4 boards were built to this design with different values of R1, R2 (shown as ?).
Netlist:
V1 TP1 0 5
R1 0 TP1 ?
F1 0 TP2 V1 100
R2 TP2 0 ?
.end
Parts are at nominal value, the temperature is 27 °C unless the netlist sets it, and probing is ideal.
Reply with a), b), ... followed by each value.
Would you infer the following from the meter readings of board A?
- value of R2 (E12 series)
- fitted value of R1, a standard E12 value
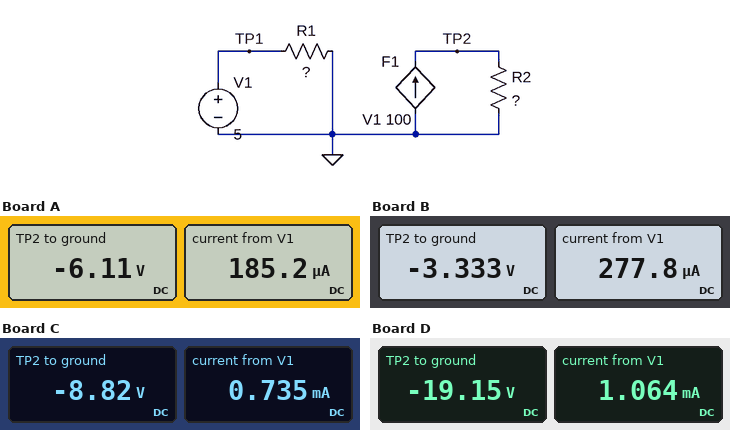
a) 330 Ω
b) 27 kΩ
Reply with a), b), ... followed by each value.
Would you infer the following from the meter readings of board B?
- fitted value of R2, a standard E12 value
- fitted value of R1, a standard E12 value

a) 120 Ω
b) 18 kΩ
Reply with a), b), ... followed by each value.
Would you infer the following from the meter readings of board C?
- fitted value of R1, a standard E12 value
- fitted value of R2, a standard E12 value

a) 6.8 kΩ
b) 120 Ω
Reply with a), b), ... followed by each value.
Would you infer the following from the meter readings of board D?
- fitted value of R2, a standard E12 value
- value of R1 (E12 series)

a) 180 Ω
b) 4.7 kΩ
